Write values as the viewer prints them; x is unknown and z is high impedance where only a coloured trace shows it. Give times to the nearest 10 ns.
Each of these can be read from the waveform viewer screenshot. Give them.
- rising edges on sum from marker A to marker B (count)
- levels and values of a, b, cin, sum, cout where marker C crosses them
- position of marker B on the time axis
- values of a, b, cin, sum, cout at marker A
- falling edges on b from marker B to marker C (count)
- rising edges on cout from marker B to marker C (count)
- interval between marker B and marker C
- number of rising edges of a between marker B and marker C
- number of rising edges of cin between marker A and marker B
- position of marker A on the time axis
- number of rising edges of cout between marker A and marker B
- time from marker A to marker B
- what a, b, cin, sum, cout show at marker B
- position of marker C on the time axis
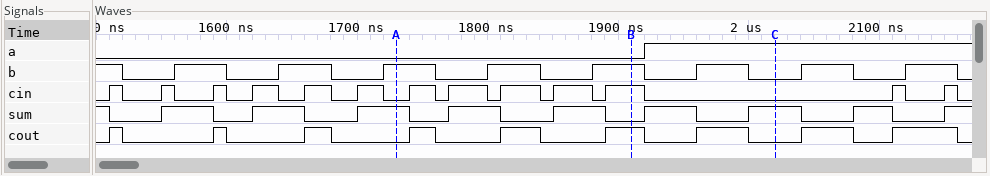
2
a=1, b=0, cin=0, sum=1, cout=0
1910 ns
a=0, b=1, cin=0, sum=1, cout=0
2
1
110 ns
1
5
1730 ns
3
180 ns
a=0, b=1, cin=1, sum=0, cout=1
2020 ns
